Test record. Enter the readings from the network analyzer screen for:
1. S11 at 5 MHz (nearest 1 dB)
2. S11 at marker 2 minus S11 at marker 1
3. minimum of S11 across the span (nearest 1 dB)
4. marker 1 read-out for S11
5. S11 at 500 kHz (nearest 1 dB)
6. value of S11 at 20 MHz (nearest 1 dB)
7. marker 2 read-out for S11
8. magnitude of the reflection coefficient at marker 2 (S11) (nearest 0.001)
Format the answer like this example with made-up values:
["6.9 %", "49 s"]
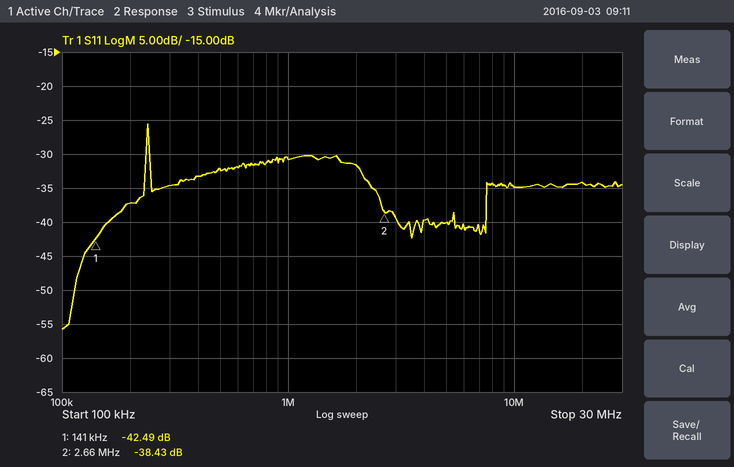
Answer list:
["-40 dB", "4.06 dB", "-56 dB", "-42.49 dB", "-32 dB", "-34 dB", "-38.43 dB", "0.012"]
